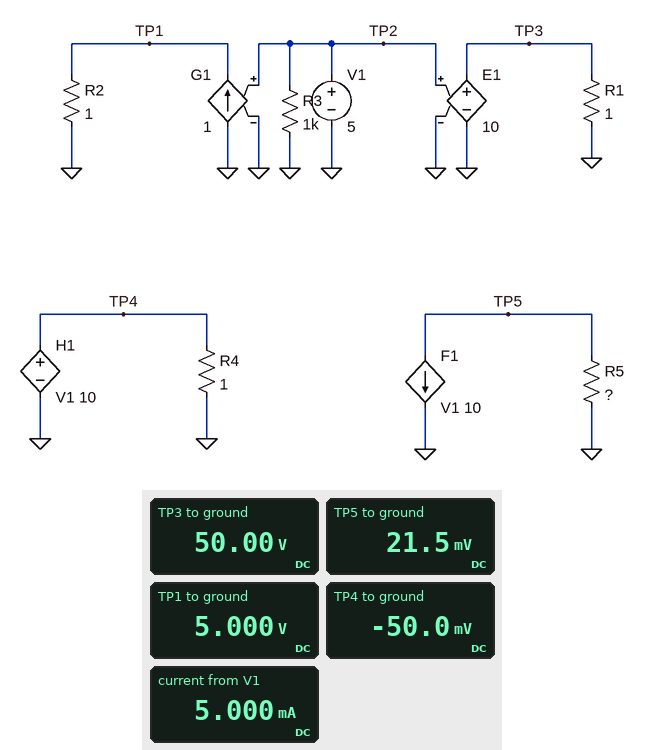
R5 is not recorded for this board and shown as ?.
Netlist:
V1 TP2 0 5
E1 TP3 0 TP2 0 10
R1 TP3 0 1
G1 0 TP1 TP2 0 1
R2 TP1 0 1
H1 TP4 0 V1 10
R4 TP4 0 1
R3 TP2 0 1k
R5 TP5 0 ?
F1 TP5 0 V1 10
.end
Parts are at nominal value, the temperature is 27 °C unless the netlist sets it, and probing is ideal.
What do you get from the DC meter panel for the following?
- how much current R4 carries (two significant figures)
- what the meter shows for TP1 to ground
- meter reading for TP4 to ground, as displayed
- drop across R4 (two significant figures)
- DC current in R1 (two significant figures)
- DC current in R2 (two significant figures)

50 mA
5.000 V
-50.0 mV
50 mV
50 A
5.0 A
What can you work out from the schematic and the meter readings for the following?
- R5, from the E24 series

0.43 Ω
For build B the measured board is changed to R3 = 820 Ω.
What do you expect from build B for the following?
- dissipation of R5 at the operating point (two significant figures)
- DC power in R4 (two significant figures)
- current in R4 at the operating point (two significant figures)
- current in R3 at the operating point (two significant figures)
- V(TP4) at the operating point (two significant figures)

1.6 mW
3.7 mW
61 mA
6.1 mA
-61 mV
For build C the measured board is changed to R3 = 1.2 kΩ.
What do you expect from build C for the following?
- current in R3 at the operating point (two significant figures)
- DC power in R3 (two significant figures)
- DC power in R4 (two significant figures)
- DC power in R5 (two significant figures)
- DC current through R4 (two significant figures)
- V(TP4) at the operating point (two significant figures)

4.2 mA
21 mW
1.7 mW
750 µW
42 mA
-42 mV
